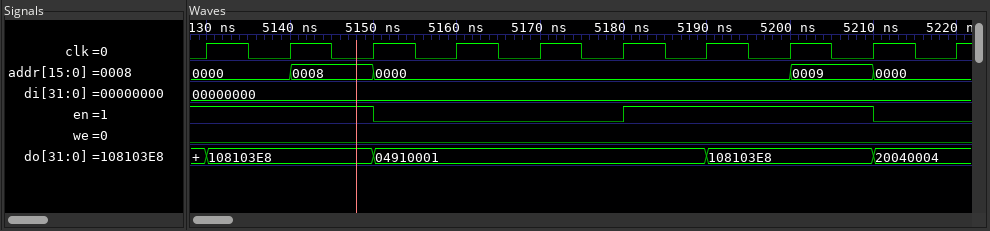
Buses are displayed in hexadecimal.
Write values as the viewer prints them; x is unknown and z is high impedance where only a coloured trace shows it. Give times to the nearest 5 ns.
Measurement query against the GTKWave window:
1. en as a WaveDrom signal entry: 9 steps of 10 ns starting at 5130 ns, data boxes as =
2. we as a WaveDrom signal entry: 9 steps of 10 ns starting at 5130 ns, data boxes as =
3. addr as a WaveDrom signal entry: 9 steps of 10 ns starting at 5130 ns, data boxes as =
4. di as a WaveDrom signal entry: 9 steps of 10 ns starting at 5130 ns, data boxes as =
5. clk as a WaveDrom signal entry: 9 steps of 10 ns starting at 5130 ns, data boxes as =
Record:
{name: 'en', wave: '1.0..1..0'}
{name: 'we', wave: '0........'}
{name: 'addr', wave: '===....==', data: '0000 0008 0000 0009 0000'}
{name: 'di', wave: '=........', data: '00000000'}
{name: 'clk', wave: 'p........'}
